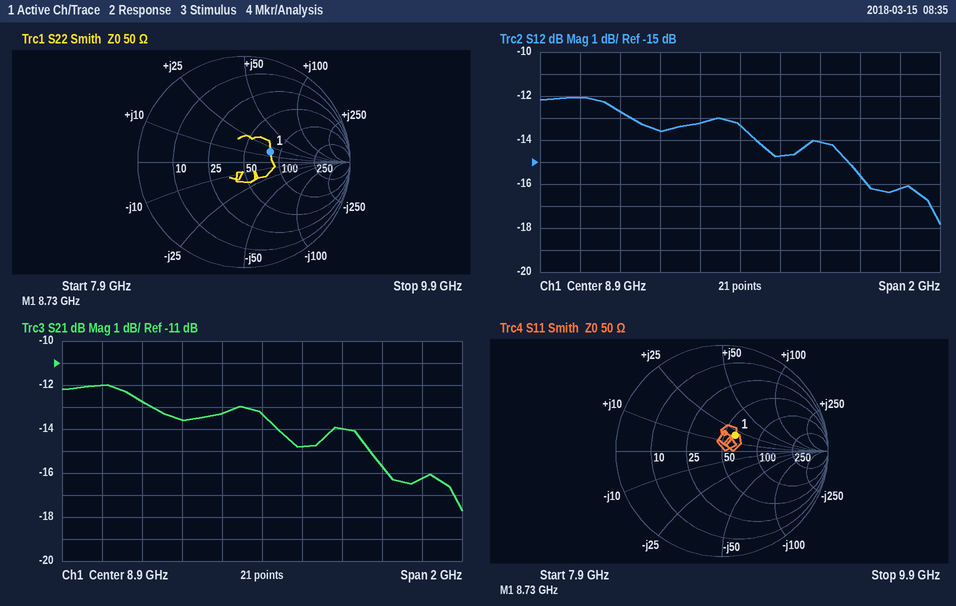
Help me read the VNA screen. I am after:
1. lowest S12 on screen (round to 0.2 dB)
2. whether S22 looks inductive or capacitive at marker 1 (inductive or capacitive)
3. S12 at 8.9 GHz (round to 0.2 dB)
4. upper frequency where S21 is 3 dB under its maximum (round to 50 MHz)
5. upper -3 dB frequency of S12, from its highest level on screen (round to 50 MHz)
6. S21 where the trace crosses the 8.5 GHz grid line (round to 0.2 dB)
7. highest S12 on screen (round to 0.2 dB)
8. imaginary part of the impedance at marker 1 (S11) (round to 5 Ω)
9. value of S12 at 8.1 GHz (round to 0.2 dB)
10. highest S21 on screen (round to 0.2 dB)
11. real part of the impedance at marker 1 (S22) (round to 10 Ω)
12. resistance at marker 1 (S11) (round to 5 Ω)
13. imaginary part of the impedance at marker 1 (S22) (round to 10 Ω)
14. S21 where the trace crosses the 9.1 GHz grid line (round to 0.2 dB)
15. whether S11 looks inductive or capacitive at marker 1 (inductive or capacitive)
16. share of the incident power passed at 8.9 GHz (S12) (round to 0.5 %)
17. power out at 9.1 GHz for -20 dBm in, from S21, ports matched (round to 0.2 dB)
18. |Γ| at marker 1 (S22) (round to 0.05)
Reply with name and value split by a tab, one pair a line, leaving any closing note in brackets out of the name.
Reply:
lowest S12 on screen	-17.8 dB
whether S22 looks inductive or capacitive at marker 1	inductive
S12 at 8.9 GHz	-13.4 dB
upper frequency where S21 is 3 dB under its maximum	9.45 GHz
upper -3 dB frequency of S12, from its highest level on screen	9.45 GHz
S21 where the trace crosses the 8.5 GHz grid line	-13.6 dB
highest S12 on screen	-12.0 dB
imaginary part of the impedance at marker 1 (S11)	+20 Ω
value of S12 at 8.1 GHz	-12.0 dB
highest S21 on screen	-12.0 dB
real part of the impedance at marker 1 (S22)	80 Ω
resistance at marker 1 (S11)	60 Ω
imaginary part of the impedance at marker 1 (S22)	+20 Ω
S21 where the trace crosses the 9.1 GHz grid line	-14.8 dB
whether S11 looks inductive or capacitive at marker 1	inductive
share of the incident power passed at 8.9 GHz (S12)	4.5 %
power out at 9.1 GHz for -20 dBm in, from S21, ports matched	-34.8 dBm
|Γ| at marker 1 (S22)	0.25
